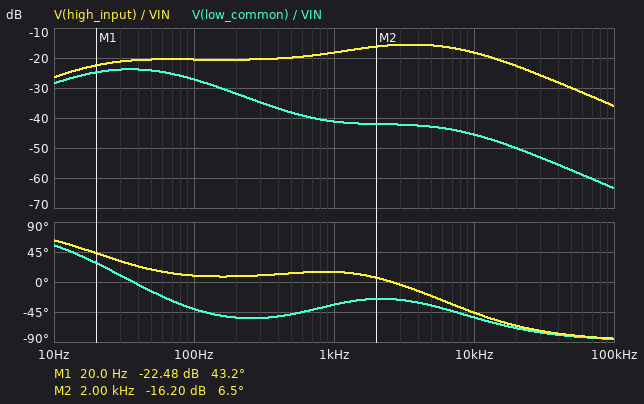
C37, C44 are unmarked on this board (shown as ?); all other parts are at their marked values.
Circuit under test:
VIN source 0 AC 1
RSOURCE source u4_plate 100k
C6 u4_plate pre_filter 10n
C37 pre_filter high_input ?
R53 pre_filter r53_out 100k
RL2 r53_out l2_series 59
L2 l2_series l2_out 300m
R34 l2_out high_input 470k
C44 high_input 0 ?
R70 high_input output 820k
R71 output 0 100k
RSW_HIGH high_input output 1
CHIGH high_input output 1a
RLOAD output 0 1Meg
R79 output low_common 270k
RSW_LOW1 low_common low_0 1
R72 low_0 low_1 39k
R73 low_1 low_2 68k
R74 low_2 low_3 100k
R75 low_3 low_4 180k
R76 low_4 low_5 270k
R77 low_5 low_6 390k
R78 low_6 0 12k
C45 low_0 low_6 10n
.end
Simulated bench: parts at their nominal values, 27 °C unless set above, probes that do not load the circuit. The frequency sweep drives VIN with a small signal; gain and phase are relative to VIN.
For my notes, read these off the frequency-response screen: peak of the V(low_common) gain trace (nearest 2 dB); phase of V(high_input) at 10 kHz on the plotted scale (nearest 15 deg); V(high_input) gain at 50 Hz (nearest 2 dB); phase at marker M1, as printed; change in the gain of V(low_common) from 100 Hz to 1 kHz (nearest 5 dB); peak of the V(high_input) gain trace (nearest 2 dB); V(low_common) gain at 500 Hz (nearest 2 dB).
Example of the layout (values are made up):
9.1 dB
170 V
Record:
-24 dB
-45 deg
-20 dB
43.2 deg
-15 dB
-16 dB
-38 dB
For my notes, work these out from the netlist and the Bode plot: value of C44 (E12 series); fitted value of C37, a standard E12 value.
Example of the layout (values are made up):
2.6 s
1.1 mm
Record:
1 nF
330 pF
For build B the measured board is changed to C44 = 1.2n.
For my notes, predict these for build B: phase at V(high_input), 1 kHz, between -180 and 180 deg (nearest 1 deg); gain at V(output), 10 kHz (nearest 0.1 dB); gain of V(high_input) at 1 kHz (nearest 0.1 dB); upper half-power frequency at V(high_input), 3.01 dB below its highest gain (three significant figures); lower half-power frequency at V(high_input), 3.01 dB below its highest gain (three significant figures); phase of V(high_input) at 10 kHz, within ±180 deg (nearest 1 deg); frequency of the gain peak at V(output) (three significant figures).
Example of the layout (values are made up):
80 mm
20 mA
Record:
12 deg
-19.5 dB
-18.5 dB
9.85 kHz
660 Hz
-49 deg
3.15 kHz
